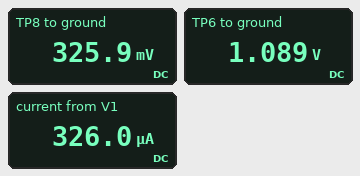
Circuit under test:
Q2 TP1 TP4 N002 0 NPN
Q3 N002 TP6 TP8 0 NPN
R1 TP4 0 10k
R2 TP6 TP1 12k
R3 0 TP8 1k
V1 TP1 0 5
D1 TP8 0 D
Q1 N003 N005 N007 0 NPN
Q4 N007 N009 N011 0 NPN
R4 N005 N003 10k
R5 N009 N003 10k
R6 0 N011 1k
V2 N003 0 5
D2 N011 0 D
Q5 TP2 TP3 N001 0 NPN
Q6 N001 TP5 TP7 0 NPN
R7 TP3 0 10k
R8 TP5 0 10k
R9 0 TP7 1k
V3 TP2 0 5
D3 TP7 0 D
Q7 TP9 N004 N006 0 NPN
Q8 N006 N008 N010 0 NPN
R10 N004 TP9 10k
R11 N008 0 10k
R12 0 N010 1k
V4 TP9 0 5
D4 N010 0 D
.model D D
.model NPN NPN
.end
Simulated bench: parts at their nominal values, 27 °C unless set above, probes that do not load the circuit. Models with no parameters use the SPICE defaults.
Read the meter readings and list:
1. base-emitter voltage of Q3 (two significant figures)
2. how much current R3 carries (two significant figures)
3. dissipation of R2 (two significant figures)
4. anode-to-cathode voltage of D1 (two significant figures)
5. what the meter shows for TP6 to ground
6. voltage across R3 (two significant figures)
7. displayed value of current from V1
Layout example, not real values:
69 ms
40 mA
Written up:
760 mV
330 µA
1.3 mW
330 mV
1.089 V
330 mV
326.0 µA
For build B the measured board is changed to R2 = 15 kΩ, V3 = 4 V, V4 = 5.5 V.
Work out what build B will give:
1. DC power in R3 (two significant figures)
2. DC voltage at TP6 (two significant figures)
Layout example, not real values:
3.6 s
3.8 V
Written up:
70 µW
1.0 V
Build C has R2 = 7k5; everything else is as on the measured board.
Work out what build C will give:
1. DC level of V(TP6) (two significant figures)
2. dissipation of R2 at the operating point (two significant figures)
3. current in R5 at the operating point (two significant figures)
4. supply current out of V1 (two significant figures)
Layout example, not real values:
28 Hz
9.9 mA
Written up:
1.3 V
1.9 mW
340 µA
500 µA
